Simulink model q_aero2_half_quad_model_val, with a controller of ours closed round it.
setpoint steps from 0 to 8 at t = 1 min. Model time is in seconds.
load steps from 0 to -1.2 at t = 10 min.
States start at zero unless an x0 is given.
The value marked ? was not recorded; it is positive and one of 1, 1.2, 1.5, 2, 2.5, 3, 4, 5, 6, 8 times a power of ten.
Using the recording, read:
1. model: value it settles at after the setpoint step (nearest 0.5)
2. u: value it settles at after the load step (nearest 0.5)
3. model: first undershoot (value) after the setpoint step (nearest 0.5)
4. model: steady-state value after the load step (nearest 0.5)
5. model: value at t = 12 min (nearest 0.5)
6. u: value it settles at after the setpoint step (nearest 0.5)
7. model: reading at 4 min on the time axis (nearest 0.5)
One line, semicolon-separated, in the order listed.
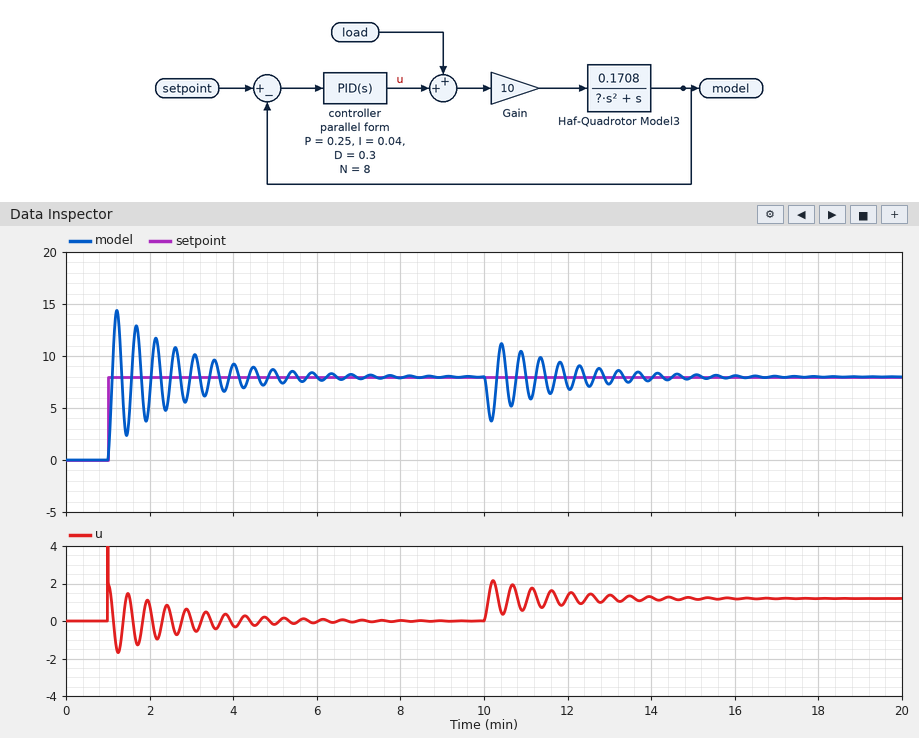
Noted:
8.0; 1.0; 2.5; 8.0; 7.0; 0.0; 9.0
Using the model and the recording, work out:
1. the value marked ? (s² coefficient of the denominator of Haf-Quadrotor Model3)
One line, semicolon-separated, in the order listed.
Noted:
8
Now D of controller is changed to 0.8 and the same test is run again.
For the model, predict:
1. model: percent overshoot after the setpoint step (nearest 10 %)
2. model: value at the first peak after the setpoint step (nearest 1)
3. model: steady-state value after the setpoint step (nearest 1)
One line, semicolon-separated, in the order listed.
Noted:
50 %; 12; 8
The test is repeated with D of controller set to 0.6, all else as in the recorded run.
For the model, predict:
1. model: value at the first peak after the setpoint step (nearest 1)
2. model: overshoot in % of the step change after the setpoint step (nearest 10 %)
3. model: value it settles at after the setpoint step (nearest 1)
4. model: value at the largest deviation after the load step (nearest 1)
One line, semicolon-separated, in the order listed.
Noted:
13; 60 %; 8; 4
